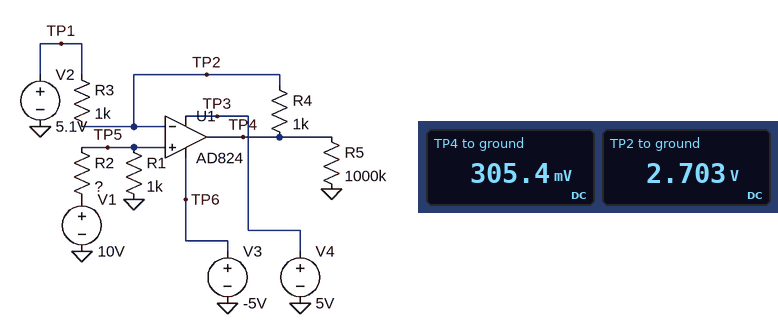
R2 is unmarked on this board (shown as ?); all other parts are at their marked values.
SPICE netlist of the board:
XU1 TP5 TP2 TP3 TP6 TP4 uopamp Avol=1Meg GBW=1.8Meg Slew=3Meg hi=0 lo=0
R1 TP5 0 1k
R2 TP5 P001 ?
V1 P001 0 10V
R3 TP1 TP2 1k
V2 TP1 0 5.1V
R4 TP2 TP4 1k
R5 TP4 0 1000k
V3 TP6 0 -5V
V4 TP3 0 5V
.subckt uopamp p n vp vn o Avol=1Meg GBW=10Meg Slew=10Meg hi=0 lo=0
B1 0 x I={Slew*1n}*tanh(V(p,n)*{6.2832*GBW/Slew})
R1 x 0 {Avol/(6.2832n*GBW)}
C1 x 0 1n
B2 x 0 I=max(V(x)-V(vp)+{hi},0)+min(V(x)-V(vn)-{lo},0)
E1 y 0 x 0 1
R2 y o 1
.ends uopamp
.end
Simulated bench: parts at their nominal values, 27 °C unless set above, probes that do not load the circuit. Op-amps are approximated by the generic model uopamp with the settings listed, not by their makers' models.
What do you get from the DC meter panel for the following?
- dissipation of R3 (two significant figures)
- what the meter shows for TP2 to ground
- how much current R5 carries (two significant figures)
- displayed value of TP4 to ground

5.7 mW
2.703 V
310 nA
305.4 mV
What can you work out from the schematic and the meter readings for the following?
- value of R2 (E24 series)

2.7 kΩ
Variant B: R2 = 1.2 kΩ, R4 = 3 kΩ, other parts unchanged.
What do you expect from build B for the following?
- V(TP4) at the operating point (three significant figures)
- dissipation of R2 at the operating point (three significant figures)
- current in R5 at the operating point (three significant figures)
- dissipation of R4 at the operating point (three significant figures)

2.88 V
24.8 mW
2.88 µA
923 µW
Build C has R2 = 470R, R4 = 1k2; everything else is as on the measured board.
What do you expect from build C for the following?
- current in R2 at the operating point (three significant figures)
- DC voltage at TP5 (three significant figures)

6.80 mA
6.80 V
